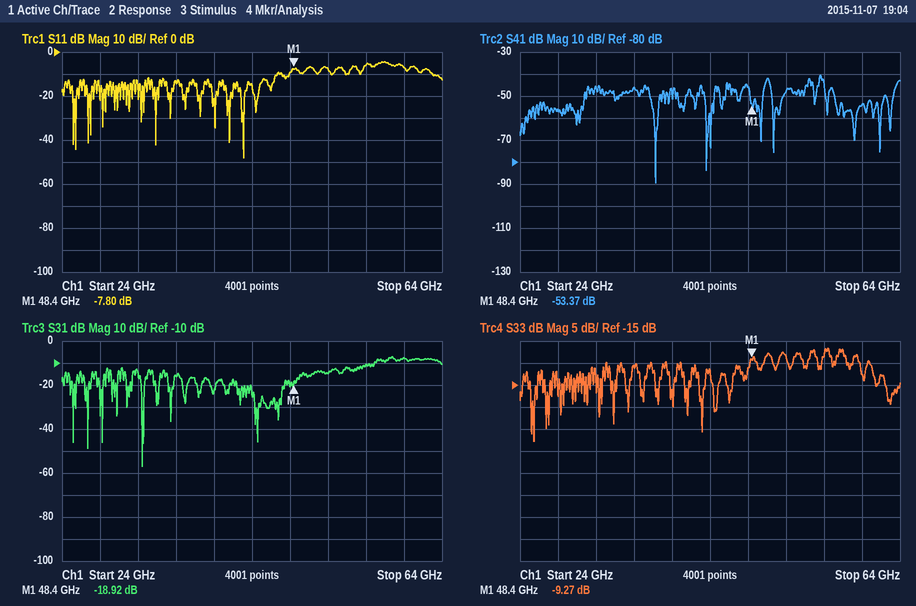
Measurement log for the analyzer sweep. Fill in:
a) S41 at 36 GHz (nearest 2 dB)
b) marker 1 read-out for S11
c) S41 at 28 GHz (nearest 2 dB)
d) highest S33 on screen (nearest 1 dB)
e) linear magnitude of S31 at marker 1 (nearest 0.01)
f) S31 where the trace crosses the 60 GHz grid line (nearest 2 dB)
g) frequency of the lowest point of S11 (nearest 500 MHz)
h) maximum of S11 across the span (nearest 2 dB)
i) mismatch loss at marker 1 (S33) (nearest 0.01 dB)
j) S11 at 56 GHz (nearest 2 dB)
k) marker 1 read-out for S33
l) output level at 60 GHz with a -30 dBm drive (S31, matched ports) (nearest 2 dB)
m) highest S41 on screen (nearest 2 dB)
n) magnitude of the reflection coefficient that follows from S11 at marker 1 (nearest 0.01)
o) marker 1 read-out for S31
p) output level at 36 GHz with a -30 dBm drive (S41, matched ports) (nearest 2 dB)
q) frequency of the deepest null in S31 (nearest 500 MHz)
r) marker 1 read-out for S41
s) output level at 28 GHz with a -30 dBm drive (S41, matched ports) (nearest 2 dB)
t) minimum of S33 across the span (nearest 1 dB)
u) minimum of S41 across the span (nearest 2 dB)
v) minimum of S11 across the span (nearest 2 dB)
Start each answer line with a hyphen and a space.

- -46 dB
- -7.80 dB
- -56 dB
- -7 dB
- 0.11
- -8 dB
- 43.0 GHz
- -4 dB
- 0.55 dB
- -6 dB
- -9.27 dB
- -38 dBm
- -40 dB
- 0.41
- -18.92 dB
- -76 dBm
- 32.5 GHz
- -53.37 dB
- -86 dBm
- -28 dB
- -90 dB
- -48 dB
